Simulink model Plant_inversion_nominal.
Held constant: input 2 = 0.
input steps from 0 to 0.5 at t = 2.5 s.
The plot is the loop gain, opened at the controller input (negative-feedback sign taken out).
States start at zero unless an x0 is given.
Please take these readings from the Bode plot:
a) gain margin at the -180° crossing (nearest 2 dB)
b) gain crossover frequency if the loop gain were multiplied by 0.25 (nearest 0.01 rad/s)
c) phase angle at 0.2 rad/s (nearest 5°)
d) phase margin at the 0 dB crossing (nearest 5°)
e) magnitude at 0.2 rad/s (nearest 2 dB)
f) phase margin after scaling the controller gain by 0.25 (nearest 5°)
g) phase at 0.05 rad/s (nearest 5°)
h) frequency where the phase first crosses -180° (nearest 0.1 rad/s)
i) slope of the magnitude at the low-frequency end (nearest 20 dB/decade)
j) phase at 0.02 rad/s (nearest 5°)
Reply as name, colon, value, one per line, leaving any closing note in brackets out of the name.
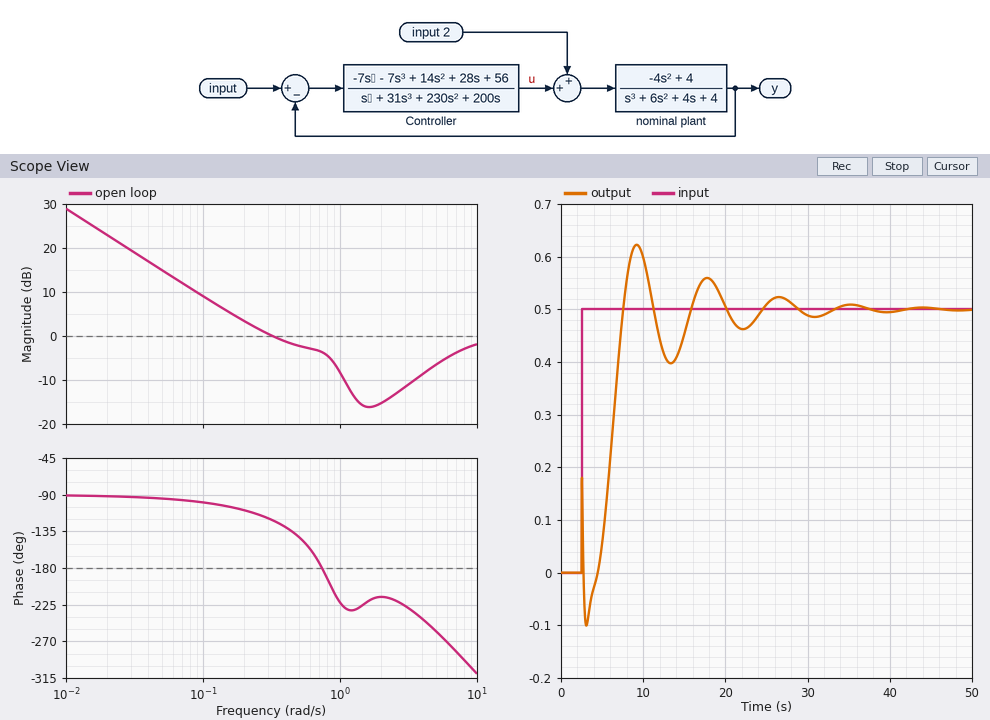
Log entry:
gain margin at the -180° crossing: 4 dB
gain crossover frequency if the loop gain were multiplied by 0.25: 0.07 rad/s
phase angle at 0.2 rad/s: -110°
phase margin at the 0 dB crossing: 60°
magnitude at 0.2 rad/s: 4 dB
phase margin after scaling the controller gain by 0.25: 85°
phase at 0.05 rad/s: -95°
frequency where the phase first crosses -180°: 0.7 rad/s
slope of the magnitude at the low-frequency end: -20 dB/decade
phase at 0.02 rad/s: -90°
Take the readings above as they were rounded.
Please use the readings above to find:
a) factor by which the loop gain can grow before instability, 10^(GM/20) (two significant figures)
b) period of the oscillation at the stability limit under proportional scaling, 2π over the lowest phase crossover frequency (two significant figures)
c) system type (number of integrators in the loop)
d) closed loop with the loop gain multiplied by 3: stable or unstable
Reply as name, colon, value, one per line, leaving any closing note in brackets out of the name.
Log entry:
factor by which the loop gain can grow before instability, 10^(GM/20): 1.6
period of the oscillation at the stability limit under proportional scaling, 2π over the lowest phase crossover frequency: 9.0 s
system type: 1
closed loop with the loop gain multiplied by 3: stable or unstable: unstable
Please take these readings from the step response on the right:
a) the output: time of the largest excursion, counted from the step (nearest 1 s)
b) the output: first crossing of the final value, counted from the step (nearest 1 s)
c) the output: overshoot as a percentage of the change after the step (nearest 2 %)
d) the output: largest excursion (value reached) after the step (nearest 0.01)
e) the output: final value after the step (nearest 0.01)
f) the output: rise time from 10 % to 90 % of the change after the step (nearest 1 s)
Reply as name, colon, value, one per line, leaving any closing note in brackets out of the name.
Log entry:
the output: time of the largest excursion, counted from the step: 7 s
the output: first crossing of the final value, counted from the step: 5 s
the output: overshoot as a percentage of the change after the step: 24 %
the output: largest excursion (value reached) after the step: 0.62
the output: final value after the step: 0.50
the output: rise time from 10 % to 90 % of the change after the step: 5 s
